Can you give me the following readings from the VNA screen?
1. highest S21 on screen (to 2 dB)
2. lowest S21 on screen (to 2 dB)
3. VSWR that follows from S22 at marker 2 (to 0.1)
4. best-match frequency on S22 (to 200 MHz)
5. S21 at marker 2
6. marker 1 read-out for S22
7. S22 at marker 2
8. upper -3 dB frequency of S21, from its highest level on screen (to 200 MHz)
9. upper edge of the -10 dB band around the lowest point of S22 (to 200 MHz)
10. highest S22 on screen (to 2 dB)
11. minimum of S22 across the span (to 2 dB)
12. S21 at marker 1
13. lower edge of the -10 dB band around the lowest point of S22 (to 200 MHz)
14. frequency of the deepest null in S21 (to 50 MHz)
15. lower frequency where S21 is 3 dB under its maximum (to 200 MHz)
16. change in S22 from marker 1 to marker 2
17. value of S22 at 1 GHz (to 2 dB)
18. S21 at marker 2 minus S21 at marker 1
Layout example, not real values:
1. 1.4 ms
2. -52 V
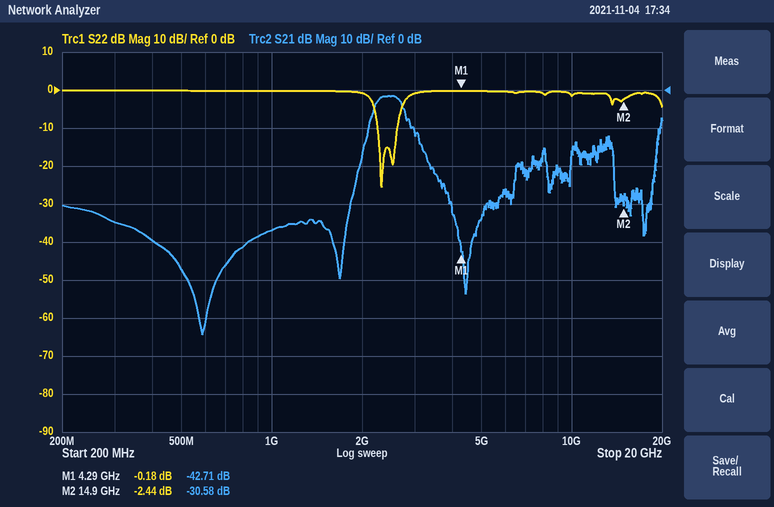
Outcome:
1. -2 dB
2. -64 dB
3. 7.2
4. 2.4 GHz
5. -30.58 dB
6. -0.18 dB
7. -2.44 dB
8. 2.8 GHz
9. 2.6 GHz
10. 0 dB
11. -26 dB
12. -42.71 dB
13. 2.2 GHz
14. 600 MHz
15. 2.2 GHz
16. -2.26 dB
17. 0 dB
18. 12.13 dB
